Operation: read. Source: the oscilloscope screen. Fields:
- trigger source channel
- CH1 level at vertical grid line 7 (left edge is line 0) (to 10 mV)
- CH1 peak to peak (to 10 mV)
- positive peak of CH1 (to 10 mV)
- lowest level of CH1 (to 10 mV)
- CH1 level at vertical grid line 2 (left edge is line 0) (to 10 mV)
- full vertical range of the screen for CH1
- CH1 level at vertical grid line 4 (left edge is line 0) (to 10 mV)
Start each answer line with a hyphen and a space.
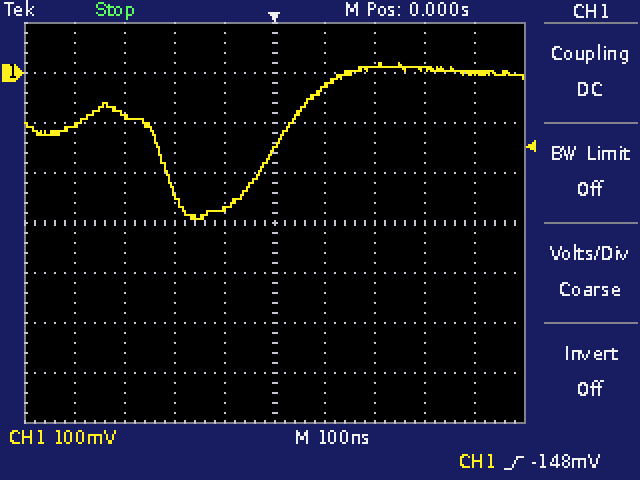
- CH1
- 10 mV
- 310 mV
- 20 mV
- -290 mV
- -80 mV
- 800 mV
- -270 mV
